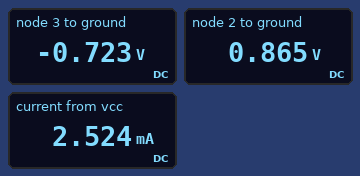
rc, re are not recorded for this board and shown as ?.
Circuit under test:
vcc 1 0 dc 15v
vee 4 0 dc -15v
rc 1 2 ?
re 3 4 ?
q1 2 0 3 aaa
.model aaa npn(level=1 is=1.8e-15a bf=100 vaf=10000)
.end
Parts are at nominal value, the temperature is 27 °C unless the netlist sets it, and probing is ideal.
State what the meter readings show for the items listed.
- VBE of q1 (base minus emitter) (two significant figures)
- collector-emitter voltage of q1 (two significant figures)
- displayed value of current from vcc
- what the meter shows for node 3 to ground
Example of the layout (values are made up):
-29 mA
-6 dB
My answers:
720 mV
1.6 V
2.524 mA
-0.723 V
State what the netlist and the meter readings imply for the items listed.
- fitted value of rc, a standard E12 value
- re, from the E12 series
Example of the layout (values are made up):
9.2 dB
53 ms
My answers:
5.6 kΩ
5.6 kΩ
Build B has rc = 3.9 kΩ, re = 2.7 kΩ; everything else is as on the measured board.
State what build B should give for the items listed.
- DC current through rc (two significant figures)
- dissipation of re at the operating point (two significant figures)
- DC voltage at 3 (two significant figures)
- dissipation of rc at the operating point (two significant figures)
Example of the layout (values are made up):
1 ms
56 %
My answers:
4.0 mA
75 mW
-750 mV
63 mW
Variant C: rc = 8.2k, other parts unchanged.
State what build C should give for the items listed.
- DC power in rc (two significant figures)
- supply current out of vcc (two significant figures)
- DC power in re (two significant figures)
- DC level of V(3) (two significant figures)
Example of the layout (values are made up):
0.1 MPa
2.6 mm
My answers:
30 mW
1.9 mA
36 mW
-730 mV
